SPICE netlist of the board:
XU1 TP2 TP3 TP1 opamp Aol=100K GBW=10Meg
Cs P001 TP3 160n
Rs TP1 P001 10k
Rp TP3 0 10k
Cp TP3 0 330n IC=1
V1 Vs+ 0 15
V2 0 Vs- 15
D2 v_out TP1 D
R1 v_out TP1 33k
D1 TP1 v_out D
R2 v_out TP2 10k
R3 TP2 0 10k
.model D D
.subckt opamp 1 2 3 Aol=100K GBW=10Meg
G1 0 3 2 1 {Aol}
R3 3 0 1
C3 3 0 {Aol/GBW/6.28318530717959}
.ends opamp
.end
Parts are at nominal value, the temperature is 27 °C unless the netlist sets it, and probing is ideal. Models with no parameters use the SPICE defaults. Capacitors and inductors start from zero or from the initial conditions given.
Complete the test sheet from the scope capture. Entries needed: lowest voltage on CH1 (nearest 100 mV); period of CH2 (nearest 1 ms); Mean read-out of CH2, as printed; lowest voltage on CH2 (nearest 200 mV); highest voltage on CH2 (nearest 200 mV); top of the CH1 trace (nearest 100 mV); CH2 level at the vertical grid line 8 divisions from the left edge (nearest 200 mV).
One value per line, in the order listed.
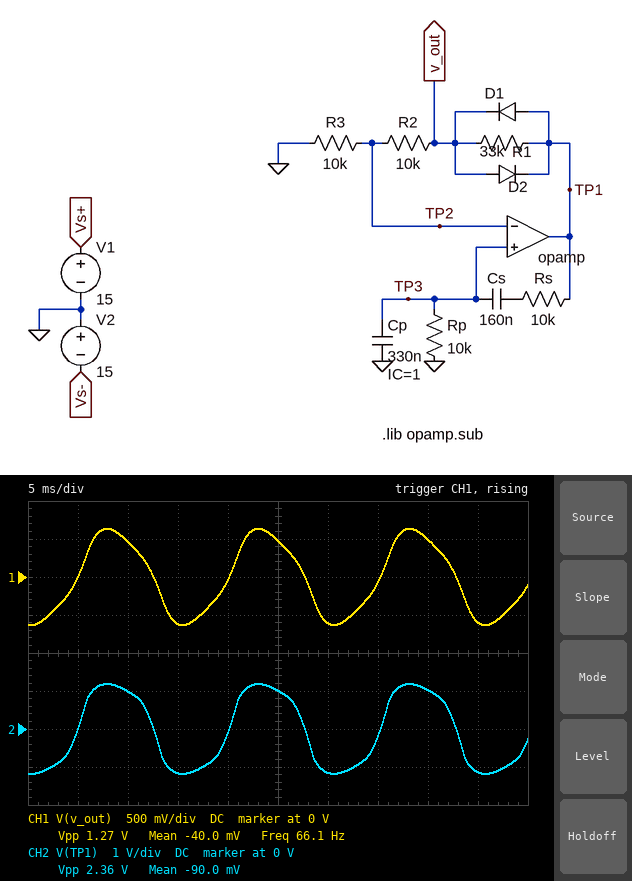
-600 mV
15 ms
-90.0 mV
-1.2 V
1.2 V
600 mV
1.0 V
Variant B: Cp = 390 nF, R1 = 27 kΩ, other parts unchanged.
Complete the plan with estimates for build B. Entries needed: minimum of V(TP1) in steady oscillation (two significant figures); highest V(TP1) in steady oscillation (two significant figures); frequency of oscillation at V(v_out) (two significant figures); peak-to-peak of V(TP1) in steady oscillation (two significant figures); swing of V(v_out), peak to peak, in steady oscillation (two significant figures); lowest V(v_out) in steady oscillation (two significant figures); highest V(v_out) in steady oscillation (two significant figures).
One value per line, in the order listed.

-970 mV
970 mV
63 Hz
1.9 V
910 mV
-460 mV
460 mV
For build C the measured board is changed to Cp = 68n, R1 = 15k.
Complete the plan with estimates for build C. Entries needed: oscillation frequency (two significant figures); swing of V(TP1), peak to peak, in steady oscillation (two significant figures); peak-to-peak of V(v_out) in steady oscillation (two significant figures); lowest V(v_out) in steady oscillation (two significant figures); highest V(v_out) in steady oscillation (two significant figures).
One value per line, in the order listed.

150 Hz
8.3 V
7.1 V
-3.5 V
3.5 V
